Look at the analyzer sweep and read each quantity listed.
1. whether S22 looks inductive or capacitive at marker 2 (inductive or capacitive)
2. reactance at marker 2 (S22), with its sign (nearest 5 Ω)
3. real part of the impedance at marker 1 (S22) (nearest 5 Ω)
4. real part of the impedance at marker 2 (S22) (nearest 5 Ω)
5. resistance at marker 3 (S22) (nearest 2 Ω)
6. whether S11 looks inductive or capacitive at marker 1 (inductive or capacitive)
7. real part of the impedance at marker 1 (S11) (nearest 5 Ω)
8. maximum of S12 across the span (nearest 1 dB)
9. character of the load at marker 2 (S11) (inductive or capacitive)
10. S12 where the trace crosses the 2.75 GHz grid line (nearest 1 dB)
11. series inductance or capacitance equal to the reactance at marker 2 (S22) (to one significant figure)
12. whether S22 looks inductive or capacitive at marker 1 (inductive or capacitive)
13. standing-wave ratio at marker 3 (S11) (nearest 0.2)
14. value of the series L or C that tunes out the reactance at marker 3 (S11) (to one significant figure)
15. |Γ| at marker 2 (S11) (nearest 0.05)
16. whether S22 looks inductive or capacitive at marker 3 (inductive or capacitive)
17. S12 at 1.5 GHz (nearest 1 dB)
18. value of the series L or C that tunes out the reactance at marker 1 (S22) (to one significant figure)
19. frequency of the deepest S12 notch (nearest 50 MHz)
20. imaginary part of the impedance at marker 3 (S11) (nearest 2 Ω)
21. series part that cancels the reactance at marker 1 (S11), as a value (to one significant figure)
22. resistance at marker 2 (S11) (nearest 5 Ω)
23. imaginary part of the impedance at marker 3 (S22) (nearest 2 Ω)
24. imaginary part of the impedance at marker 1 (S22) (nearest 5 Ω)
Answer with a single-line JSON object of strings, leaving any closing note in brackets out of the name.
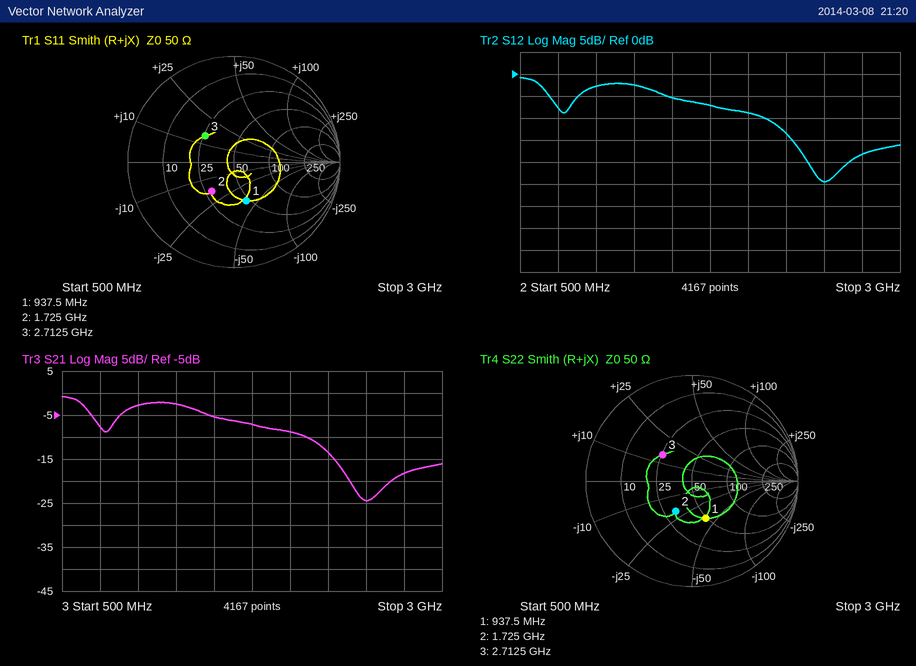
{"whether S22 looks inductive or capacitive at marker 2": "capacitive", "reactance at marker 2 (S22), with its sign": "-20 Ω", "real part of the impedance at marker 1 (S22)": "50 Ω", "real part of the impedance at marker 2 (S22)": "30 Ω", "resistance at marker 3 (S22)": "26 Ω", "whether S11 looks inductive or capacitive at marker 1": "capacitive", "real part of the impedance at marker 1 (S11)": "45 Ω", "maximum of S12 across the span": "-1 dB", "character of the load at marker 2 (S11)": "capacitive", "S12 where the trace crosses the 2.75 GHz grid line": "-18 dB", "series inductance or capacitance equal to the reactance at marker 2 (S22)": "5 pF", "whether S22 looks inductive or capacitive at marker 1": "capacitive", "standing-wave ratio at marker 3 (S11)": "2.2", "value of the series L or C that tunes out the reactance at marker 3 (S11)": "4 pF", "|Γ| at marker 2 (S11)": "0.35", "whether S22 looks inductive or capacitive at marker 3": "inductive", "S12 at 1.5 GHz": "-5 dB", "value of the series L or C that tunes out the reactance at marker 1 (S22)": "7 nH", "frequency of the deepest S12 notch": "2.50 GHz", "imaginary part of the impedance at marker 3 (S11)": "+14 Ω", "series part that cancels the reactance at marker 1 (S11), as a value": "7 nH", "resistance at marker 2 (S11)": "30 Ω", "imaginary part of the impedance at marker 3 (S22)": "+14 Ω", "imaginary part of the impedance at marker 1 (S22)": "-40 Ω"}
